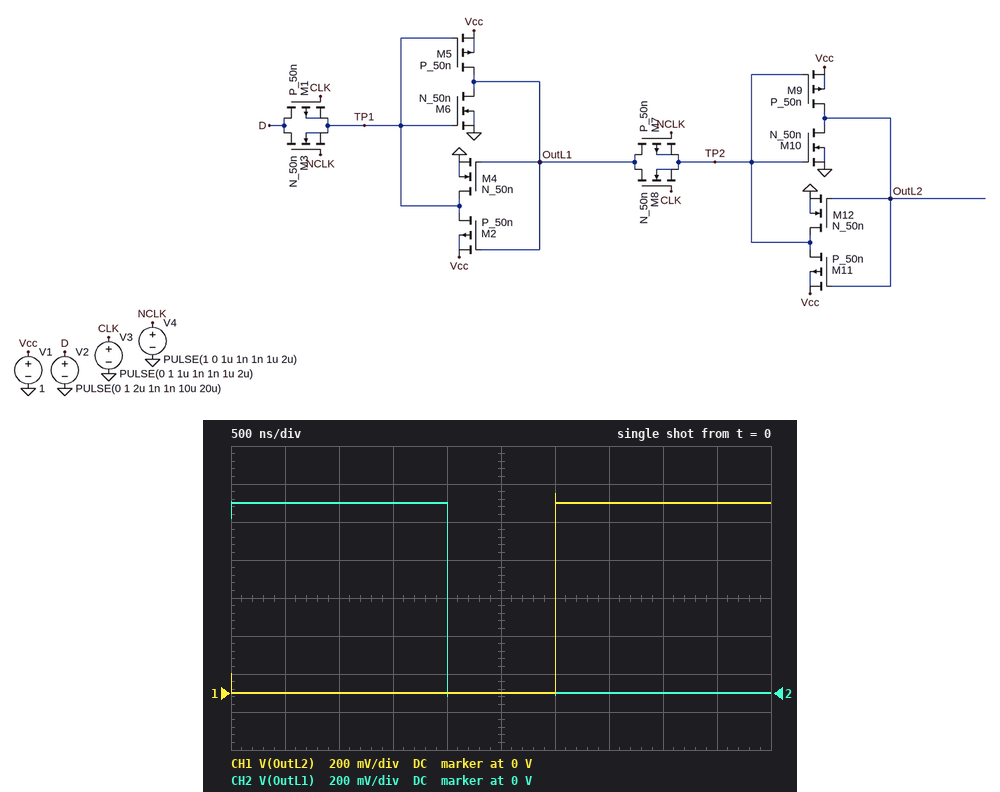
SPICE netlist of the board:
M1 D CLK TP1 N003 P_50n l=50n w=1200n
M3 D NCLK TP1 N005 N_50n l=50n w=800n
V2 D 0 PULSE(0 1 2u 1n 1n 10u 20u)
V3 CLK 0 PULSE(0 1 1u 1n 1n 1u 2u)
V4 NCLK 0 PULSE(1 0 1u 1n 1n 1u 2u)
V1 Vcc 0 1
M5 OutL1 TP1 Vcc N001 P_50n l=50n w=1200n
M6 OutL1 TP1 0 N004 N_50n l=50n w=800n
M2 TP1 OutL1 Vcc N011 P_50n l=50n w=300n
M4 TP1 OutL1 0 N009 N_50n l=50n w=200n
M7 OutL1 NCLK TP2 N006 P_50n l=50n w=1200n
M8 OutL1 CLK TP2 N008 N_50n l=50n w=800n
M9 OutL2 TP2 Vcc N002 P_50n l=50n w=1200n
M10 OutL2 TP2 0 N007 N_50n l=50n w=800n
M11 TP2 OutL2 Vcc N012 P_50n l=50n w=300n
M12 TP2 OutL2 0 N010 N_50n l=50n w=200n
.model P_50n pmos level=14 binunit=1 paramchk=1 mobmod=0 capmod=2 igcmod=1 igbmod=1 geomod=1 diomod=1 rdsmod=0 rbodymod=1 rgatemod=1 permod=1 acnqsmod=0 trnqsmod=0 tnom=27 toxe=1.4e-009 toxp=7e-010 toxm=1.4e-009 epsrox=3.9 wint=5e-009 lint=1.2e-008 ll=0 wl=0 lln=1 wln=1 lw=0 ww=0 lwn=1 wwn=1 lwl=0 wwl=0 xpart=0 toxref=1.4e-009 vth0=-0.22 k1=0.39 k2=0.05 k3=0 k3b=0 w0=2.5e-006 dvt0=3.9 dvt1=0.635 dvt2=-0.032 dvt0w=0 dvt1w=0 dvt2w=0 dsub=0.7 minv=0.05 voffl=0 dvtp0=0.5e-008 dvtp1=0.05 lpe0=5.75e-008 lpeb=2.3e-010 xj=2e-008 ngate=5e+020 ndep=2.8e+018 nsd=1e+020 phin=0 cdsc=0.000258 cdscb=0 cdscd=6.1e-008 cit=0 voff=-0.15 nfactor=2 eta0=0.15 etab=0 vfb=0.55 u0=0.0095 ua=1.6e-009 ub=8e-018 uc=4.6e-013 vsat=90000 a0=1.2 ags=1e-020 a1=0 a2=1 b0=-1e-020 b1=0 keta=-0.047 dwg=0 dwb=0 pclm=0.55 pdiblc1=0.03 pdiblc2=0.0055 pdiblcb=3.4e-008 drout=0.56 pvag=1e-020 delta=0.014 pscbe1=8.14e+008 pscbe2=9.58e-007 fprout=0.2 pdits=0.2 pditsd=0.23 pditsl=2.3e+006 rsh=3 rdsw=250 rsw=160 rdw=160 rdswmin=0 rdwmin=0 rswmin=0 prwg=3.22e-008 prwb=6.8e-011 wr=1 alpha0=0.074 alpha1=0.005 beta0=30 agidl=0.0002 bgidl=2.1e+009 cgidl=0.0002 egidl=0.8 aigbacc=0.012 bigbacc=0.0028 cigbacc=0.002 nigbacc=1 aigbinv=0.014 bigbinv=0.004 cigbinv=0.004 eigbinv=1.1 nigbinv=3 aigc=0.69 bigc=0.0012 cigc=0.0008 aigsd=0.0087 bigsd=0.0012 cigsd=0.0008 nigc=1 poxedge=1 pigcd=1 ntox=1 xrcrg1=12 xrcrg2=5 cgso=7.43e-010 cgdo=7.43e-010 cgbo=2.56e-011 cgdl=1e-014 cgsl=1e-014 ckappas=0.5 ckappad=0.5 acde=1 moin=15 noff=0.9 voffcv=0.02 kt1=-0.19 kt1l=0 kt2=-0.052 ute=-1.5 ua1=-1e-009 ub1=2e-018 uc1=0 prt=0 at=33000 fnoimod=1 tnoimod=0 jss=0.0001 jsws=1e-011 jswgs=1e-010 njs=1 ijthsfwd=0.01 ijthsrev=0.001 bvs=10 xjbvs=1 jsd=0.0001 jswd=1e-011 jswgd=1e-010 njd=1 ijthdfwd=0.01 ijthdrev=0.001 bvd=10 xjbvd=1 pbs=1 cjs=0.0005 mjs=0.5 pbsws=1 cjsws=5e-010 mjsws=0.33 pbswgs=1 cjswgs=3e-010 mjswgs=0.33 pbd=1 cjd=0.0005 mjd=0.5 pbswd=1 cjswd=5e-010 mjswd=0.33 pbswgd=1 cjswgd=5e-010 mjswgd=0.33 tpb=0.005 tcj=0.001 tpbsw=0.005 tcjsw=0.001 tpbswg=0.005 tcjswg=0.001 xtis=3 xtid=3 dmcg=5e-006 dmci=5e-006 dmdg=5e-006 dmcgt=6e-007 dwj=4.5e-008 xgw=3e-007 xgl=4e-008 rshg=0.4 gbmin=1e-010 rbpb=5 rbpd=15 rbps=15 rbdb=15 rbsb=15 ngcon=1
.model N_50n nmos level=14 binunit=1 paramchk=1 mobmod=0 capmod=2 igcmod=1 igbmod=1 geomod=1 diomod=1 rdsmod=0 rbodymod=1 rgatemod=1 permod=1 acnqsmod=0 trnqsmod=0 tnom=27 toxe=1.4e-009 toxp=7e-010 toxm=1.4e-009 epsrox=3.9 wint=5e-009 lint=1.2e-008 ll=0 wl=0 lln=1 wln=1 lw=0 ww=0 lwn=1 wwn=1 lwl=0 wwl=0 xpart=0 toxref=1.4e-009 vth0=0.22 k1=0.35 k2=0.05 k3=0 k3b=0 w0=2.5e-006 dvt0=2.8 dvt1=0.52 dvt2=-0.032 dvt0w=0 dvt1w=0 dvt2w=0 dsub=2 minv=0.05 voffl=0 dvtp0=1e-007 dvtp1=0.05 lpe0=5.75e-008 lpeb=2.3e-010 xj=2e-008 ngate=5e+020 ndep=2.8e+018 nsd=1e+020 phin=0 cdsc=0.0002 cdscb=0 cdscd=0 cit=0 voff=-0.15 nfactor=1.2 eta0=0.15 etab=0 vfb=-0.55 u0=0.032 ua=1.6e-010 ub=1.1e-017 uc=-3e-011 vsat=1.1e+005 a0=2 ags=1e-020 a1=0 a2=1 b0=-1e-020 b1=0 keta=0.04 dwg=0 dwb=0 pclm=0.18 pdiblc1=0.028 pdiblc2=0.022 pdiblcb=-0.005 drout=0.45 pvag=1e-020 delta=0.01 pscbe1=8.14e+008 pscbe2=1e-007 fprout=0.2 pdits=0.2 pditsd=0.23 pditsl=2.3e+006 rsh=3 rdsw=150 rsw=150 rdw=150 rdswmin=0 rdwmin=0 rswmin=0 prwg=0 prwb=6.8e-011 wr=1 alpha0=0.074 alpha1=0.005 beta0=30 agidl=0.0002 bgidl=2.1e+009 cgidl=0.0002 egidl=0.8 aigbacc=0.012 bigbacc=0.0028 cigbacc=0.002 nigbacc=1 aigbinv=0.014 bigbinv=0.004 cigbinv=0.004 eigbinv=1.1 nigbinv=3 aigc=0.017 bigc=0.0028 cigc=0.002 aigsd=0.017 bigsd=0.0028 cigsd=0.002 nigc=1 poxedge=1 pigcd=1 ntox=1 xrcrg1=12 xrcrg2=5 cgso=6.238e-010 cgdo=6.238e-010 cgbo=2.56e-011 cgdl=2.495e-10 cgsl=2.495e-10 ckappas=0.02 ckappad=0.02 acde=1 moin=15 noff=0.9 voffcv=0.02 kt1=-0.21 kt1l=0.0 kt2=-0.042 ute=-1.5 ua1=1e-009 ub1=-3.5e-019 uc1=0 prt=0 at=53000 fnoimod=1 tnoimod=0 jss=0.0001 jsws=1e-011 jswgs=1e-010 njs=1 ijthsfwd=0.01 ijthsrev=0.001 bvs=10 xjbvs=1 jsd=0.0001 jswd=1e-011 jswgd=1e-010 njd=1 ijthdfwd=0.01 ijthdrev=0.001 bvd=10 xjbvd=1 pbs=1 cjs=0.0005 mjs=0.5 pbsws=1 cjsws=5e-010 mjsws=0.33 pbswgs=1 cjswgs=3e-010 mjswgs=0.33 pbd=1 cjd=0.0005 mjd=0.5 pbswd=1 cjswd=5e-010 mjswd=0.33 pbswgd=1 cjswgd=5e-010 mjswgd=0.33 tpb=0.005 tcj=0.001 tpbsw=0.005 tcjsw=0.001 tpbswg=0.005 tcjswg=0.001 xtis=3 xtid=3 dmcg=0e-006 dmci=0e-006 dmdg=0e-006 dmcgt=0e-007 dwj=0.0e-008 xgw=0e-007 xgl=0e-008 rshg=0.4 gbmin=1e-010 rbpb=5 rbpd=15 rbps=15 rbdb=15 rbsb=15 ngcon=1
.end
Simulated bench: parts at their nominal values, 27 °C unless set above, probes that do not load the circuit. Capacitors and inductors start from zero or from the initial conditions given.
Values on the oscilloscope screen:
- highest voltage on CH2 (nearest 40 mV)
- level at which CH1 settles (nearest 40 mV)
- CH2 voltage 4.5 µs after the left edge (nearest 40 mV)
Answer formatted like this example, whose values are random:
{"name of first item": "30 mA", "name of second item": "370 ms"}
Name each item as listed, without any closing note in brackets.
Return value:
{"highest voltage on CH2": "1.00 V", "level at which CH1 settles": "1.00 V", "CH2 voltage 4.5 µs after the left edge": "0 V"}
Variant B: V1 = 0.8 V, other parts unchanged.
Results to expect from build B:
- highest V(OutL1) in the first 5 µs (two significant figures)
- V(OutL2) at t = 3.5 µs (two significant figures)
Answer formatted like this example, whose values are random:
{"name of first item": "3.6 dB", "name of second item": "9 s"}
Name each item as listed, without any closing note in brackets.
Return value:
{"highest V(OutL1) in the first 5 µs": "810 mV", "V(OutL2) at t = 3.5 µs": "800 mV"}
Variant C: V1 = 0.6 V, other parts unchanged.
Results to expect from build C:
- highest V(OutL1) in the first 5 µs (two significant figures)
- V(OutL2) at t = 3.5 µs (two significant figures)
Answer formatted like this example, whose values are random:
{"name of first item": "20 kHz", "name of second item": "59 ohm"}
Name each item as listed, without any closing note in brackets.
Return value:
{"highest V(OutL1) in the first 5 µs": "610 mV", "V(OutL2) at t = 3.5 µs": "600 mV"}
